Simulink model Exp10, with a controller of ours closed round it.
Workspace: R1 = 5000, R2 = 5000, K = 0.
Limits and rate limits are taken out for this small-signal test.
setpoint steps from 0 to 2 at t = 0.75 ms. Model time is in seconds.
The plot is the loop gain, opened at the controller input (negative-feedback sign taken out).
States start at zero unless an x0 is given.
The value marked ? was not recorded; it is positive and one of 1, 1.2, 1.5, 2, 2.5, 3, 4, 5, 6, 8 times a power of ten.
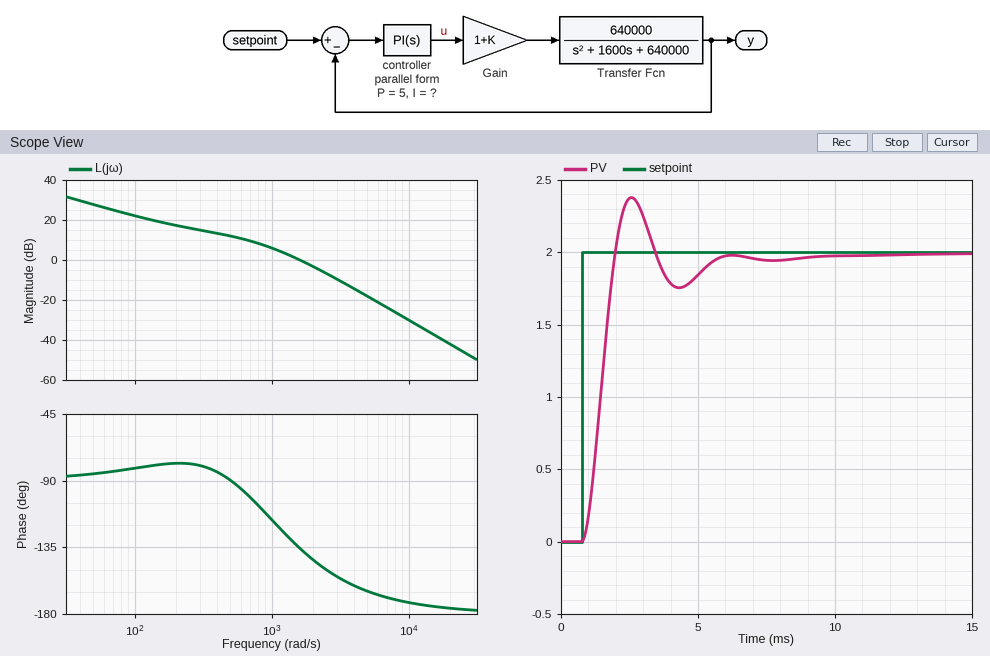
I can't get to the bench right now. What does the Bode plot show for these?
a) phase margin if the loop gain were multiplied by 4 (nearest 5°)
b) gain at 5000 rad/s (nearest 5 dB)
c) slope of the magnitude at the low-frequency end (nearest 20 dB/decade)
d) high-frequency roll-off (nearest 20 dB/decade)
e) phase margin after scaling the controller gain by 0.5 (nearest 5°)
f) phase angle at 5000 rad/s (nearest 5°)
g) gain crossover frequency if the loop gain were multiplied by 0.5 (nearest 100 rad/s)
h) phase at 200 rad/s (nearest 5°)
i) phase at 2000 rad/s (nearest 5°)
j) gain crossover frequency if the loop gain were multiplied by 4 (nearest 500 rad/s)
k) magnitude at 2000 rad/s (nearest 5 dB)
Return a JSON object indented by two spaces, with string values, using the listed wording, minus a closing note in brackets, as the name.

{
  "phase margin if the loop gain were multiplied by 4": "20°",
  "gain at 5000 rad/s": "-20 dB",
  "slope of the magnitude at the low-frequency end": "-20 dB/decade",
  "high-frequency roll-off": "-40 dB/decade",
  "phase margin after scaling the controller gain by 0.5": "65°",
  "phase angle at 5000 rad/s": "-165°",
  "gain crossover frequency if the loop gain were multiplied by 0.5": "1000 rad/s",
  "phase at 200 rad/s": "-80°",
  "phase at 2000 rad/s": "-145°",
  "gain crossover frequency if the loop gain were multiplied by 4": "3500 rad/s",
  "magnitude at 2000 rad/s": "-5 dB"
}
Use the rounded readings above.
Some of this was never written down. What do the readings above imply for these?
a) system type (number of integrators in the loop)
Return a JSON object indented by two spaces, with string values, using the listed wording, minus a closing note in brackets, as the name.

{
  "system type": "1"
}
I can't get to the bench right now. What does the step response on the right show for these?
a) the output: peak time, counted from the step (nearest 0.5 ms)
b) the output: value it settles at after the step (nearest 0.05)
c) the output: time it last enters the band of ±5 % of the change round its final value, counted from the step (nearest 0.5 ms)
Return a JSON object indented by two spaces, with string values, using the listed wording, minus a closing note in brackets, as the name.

{
  "the output: peak time, counted from the step": "2.0 ms",
  "the output: value it settles at after the step": "2.00",
  "the output: time it last enters the band of ±5 % of the change round its final value, counted from the step": "4.5 ms"
}
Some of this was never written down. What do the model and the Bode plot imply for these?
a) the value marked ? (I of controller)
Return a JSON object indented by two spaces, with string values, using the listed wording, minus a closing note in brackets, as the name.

{
  "the value marked ?": "1200"
}
